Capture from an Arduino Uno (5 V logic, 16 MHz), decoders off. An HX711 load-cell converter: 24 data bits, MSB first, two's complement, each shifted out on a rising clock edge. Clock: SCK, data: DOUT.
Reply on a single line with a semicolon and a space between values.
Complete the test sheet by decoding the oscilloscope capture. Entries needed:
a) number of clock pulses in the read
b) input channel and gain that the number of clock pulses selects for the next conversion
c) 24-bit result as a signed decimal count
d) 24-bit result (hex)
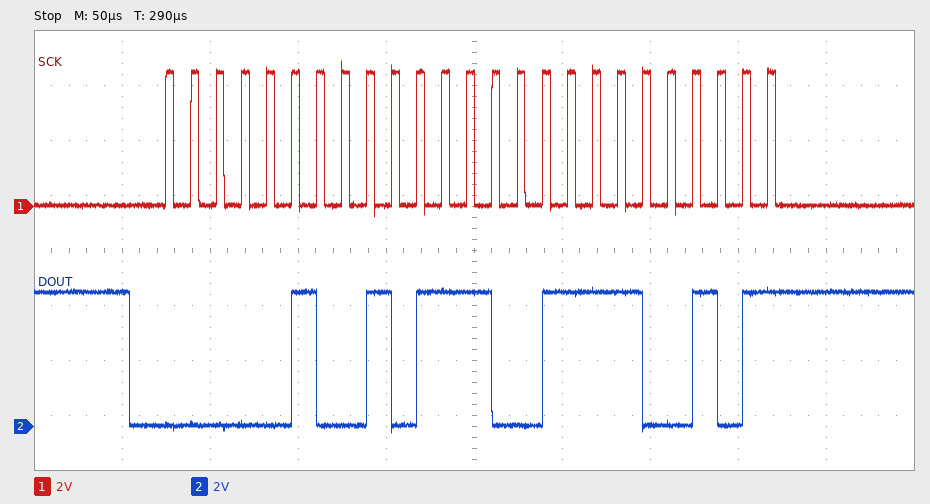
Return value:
25; channel A, gain 128; 309733; 0x04B9E5
